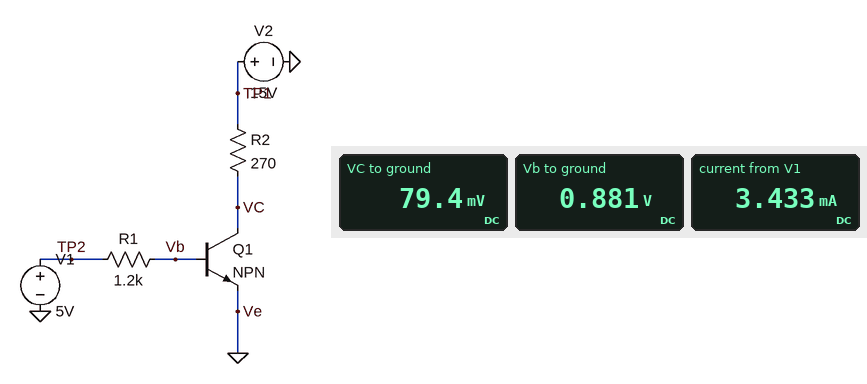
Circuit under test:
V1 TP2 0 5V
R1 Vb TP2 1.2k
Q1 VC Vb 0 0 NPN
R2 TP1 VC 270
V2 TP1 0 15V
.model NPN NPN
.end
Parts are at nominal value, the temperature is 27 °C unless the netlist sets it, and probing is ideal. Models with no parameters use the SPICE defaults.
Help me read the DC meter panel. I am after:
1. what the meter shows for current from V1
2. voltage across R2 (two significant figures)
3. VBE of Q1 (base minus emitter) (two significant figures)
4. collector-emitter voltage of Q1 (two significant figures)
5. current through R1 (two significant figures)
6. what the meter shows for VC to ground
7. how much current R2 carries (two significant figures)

3.433 mA
15 V
880 mV
79 mV
3.4 mA
79.4 mV
55 mA
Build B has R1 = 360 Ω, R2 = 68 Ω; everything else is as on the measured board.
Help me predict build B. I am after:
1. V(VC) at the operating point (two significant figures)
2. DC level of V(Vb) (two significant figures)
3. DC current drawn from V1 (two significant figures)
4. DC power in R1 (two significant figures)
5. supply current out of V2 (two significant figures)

85 mV
920 mV
11 mA
46 mW
220 mA
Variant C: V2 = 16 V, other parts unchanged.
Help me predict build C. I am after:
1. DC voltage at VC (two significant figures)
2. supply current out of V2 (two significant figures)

81 mV
59 mA
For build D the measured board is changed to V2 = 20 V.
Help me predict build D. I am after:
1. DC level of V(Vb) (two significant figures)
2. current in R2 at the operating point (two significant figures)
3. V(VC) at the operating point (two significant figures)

890 mV
74 mA
88 mV
